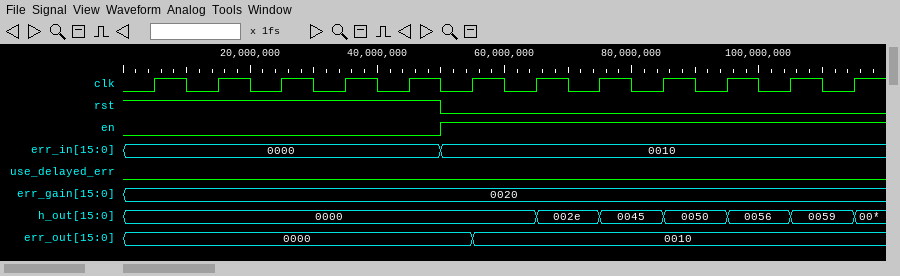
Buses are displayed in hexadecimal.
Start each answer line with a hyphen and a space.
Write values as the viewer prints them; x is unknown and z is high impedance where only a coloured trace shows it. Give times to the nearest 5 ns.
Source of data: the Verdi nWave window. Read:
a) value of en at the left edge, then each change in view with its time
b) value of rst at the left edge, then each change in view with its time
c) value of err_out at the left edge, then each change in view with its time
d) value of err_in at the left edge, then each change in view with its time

- 0, 1 at 50 ns
- 1, 0 at 50 ns
- 0000, 0010 at 55 ns
- 0000, 0010 at 50 ns
